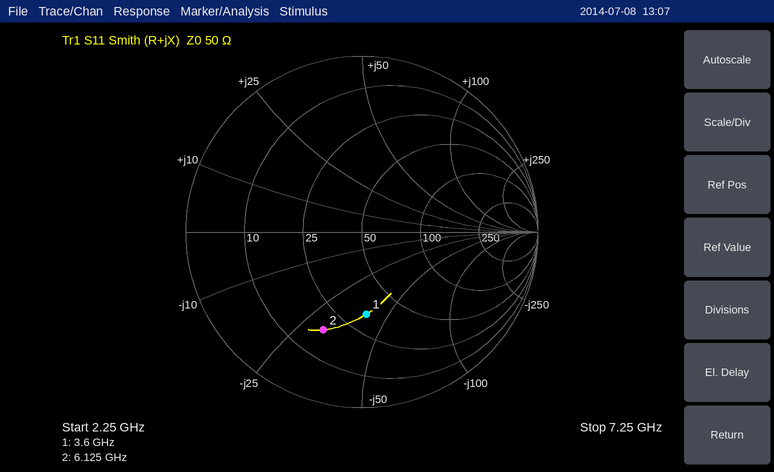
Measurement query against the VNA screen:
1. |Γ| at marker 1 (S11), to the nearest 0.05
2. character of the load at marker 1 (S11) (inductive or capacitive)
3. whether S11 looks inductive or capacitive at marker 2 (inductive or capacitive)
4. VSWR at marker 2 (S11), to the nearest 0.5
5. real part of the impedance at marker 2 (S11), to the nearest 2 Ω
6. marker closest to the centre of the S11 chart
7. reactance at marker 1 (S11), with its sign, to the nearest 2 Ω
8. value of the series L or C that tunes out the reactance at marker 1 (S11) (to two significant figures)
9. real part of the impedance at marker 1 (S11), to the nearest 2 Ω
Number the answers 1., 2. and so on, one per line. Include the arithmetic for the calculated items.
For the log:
1. 0.45
2. capacitive
3. capacitive
4. 4.0
5. 18 Ω
6. marker 1
7. -40 Ω
8. L = 40 Ω/(2π × 3.6 GHz) ≈ 1.8 nH
9. 34 Ω
